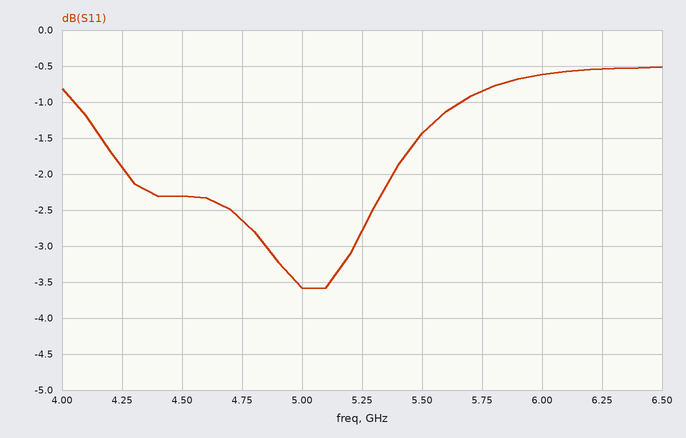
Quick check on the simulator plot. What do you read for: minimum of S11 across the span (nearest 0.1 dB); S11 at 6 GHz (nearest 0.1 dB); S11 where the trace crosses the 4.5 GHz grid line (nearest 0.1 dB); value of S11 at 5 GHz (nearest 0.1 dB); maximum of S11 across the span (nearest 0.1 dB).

-3.6 dB
-0.6 dB
-2.3 dB
-3.6 dB
-0.5 dB
